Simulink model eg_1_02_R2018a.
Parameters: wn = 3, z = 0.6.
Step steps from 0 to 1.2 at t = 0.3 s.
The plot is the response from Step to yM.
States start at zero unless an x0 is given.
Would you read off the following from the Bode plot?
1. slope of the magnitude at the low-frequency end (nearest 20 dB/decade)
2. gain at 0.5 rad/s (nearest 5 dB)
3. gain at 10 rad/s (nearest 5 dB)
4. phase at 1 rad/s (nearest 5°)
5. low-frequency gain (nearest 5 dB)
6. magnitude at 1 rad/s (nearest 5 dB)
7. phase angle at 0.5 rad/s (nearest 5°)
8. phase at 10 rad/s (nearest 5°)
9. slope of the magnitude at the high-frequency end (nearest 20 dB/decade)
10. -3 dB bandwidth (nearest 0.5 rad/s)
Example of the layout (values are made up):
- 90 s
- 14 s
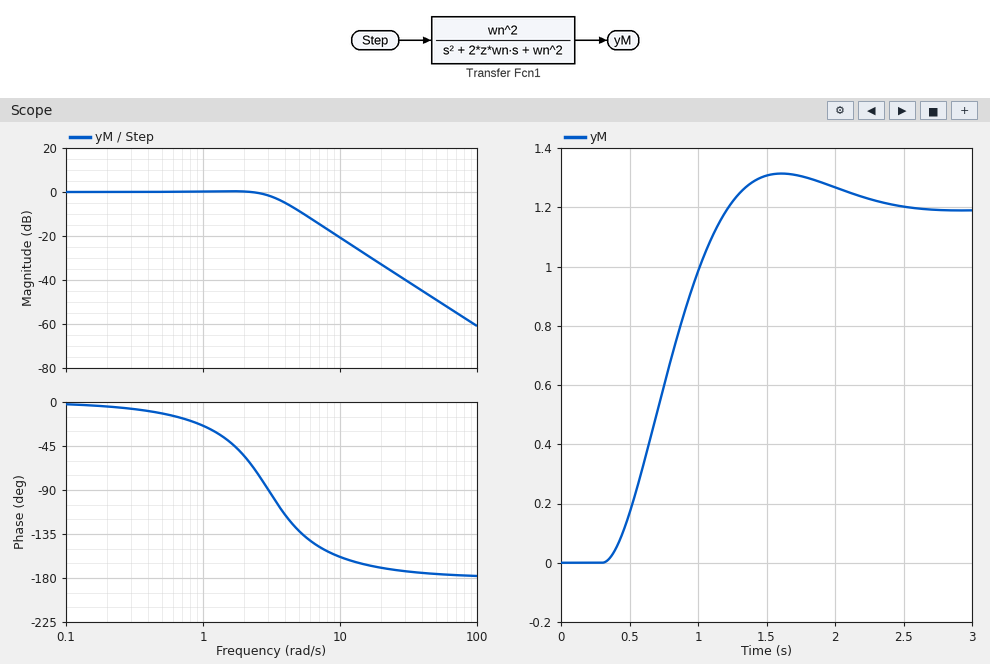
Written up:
- 0 dB/decade
- 0 dB
- -20 dB
- -25°
- 0 dB
- 0 dB
- -10°
- -160°
- -40 dB/decade
- 3.5 rad/s
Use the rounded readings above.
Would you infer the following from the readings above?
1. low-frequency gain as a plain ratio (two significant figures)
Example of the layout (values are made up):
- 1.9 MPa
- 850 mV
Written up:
- 1.0
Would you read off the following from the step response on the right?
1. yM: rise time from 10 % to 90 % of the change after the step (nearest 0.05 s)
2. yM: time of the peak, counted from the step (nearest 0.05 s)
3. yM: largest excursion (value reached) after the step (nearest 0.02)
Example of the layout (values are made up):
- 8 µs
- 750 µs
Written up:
- 0.60 s
- 1.30 s
- 1.32
